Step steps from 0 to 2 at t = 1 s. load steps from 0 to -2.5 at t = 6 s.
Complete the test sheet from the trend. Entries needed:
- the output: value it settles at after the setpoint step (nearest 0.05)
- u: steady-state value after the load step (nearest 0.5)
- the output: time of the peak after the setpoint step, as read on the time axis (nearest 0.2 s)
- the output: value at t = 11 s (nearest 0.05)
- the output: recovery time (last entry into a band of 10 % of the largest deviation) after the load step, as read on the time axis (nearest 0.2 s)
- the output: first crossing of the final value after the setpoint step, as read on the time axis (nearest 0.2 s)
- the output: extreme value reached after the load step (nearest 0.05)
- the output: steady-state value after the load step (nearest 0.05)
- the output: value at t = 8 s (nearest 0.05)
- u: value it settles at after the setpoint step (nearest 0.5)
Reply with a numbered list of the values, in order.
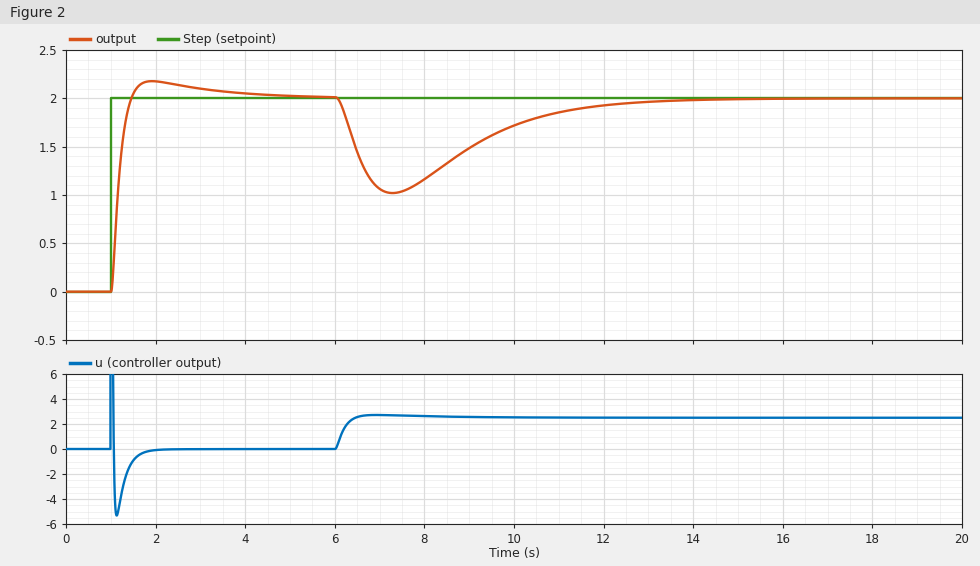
1. 2.00
2. 2.5
3. 2.0 s
4. 1.85
5. 11.6 s
6. 1.4 s
7. 1.00
8. 2.00
9. 1.15
10. 0.0
